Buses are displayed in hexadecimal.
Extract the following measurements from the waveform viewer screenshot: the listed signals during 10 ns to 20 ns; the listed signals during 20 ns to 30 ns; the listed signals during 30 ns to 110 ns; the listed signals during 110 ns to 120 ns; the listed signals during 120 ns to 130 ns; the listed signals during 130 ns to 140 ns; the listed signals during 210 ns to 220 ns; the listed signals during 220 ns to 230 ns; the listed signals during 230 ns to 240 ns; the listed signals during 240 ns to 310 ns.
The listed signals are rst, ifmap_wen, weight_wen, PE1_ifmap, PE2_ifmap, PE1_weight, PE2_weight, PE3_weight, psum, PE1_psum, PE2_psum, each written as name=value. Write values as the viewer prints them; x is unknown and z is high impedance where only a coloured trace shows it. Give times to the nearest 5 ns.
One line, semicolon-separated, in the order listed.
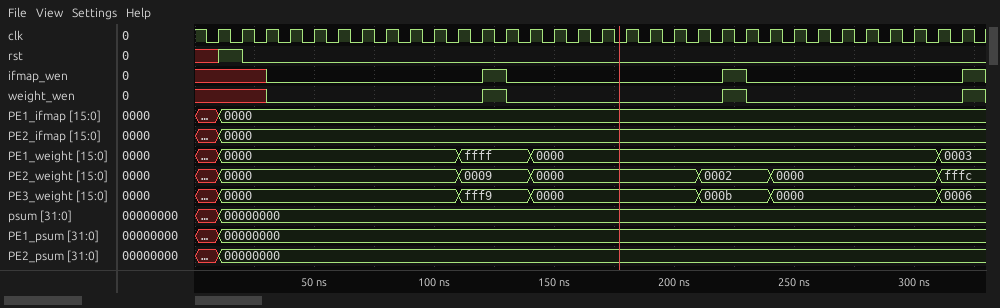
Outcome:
rst=1, ifmap_wen=x, weight_wen=x, PE1_ifmap=0000, PE2_ifmap=0000, PE1_weight=0000, PE2_weight=0000, PE3_weight=0000, psum=00000000, PE1_psum=00000000, PE2_psum=00000000; rst=0, ifmap_wen=x, weight_wen=x, PE1_ifmap=0000, PE2_ifmap=0000, PE1_weight=0000, PE2_weight=0000, PE3_weight=0000, psum=00000000, PE1_psum=00000000, PE2_psum=00000000; rst=0, ifmap_wen=0, weight_wen=0, PE1_ifmap=0000, PE2_ifmap=0000, PE1_weight=0000, PE2_weight=0000, PE3_weight=0000, psum=00000000, PE1_psum=00000000, PE2_psum=00000000; rst=0, ifmap_wen=0, weight_wen=0, PE1_ifmap=0000, PE2_ifmap=0000, PE1_weight=ffff, PE2_weight=0009, PE3_weight=fff9, psum=00000000, PE1_psum=00000000, PE2_psum=00000000; rst=0, ifmap_wen=1, weight_wen=1, PE1_ifmap=0000, PE2_ifmap=0000, PE1_weight=ffff, PE2_weight=0009, PE3_weight=fff9, psum=00000000, PE1_psum=00000000, PE2_psum=00000000; rst=0, ifmap_wen=0, weight_wen=0, PE1_ifmap=0000, PE2_ifmap=0000, PE1_weight=ffff, PE2_weight=0009, PE3_weight=fff9, psum=00000000, PE1_psum=00000000, PE2_psum=00000000; rst=0, ifmap_wen=0, weight_wen=0, PE1_ifmap=0000, PE2_ifmap=0000, PE1_weight=0000, PE2_weight=0002, PE3_weight=000b, psum=00000000, PE1_psum=00000000, PE2_psum=00000000; rst=0, ifmap_wen=1, weight_wen=1, PE1_ifmap=0000, PE2_ifmap=0000, PE1_weight=0000, PE2_weight=0002, PE3_weight=000b, psum=00000000, PE1_psum=00000000, PE2_psum=00000000; rst=0, ifmap_wen=0, weight_wen=0, PE1_ifmap=0000, PE2_ifmap=0000, PE1_weight=0000, PE2_weight=0002, PE3_weight=000b, psum=00000000, PE1_psum=00000000, PE2_psum=00000000; rst=0, ifmap_wen=0, weight_wen=0, PE1_ifmap=0000, PE2_ifmap=0000, PE1_weight=0000, PE2_weight=0000, PE3_weight=0000, psum=00000000, PE1_psum=00000000, PE2_psum=00000000
